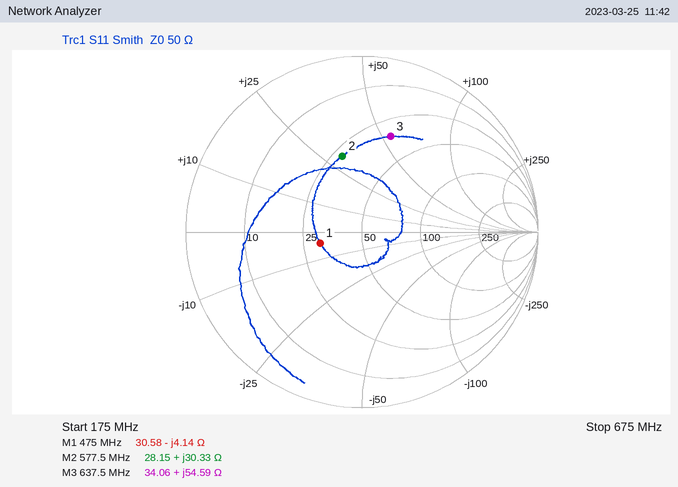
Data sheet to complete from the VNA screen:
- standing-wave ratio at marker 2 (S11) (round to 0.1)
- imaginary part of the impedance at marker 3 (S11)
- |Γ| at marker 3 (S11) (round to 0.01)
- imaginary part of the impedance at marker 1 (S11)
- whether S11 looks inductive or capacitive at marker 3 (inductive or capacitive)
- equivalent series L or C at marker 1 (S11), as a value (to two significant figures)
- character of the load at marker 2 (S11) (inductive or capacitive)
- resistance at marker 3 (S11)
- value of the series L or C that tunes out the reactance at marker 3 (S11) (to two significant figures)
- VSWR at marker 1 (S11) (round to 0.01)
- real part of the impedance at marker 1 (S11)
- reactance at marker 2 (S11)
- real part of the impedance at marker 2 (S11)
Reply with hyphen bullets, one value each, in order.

- 2.6
- +54.59 Ω
- 0.57
- -4.14 Ω
- inductive
- 81 pF
- inductive
- 34.06 Ω
- 4.6 pF
- 1.65
- 30.58 Ω
- +30.33 Ω
- 28.15 Ω
